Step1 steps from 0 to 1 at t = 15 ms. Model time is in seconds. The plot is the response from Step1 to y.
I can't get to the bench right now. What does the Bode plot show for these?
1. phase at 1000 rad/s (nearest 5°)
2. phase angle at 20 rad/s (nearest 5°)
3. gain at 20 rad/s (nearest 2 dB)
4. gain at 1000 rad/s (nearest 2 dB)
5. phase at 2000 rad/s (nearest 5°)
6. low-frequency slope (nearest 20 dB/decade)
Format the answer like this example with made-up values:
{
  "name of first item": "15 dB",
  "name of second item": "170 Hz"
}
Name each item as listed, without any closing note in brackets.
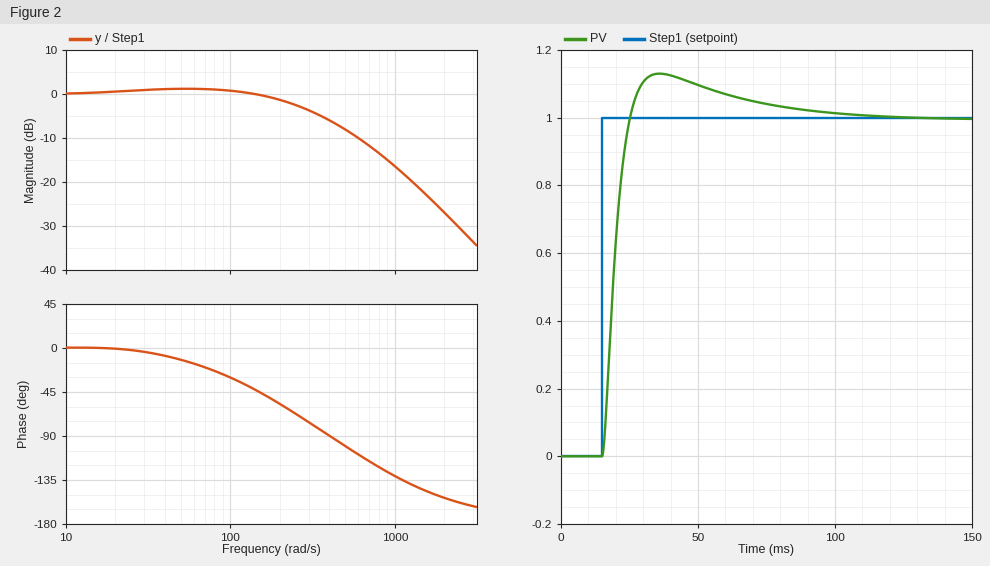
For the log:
{
  "phase at 1000 rad/s": "-130°",
  "phase angle at 20 rad/s": "0°",
  "gain at 20 rad/s": "0 dB",
  "gain at 1000 rad/s": "-16 dB",
  "phase at 2000 rad/s": "-155°",
  "low-frequency slope": "0 dB/decade"
}
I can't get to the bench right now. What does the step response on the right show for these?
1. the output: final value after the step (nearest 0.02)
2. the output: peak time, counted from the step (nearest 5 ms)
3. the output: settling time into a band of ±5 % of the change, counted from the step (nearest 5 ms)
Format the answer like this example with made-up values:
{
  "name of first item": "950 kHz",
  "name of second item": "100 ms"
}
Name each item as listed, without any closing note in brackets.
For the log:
{
  "the output: final value after the step": "1.00",
  "the output: peak time, counted from the step": "20 ms",
  "the output: settling time into a band of ±5 % of the change, counted from the step": "55 ms"
}
